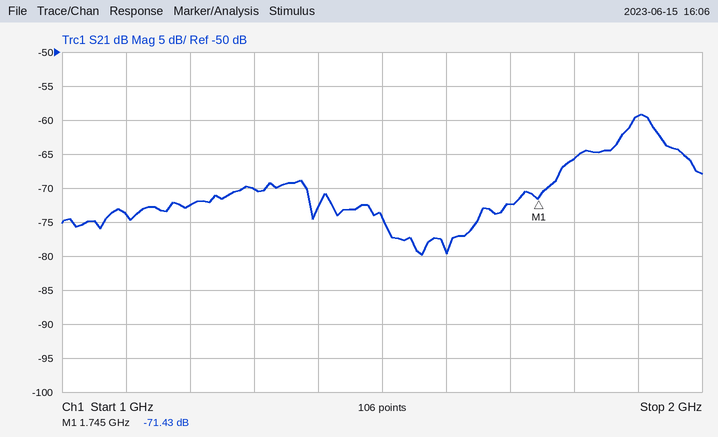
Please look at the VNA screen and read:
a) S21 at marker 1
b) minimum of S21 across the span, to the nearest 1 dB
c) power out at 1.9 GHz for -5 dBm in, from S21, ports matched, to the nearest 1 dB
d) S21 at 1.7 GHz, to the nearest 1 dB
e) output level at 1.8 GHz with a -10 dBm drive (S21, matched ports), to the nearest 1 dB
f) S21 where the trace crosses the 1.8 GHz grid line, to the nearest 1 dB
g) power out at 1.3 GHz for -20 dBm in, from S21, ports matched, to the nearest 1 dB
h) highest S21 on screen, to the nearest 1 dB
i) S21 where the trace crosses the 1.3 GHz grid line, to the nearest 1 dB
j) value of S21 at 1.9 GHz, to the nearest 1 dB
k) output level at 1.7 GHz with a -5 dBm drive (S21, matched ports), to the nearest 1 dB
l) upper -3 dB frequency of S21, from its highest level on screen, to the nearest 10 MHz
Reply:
-71.43 dB
-80 dB
-64 dBm
-72 dB
-76 dBm
-66 dB
-90 dBm
-59 dB
-70 dB
-59 dB
-77 dBm
1.93 GHz
